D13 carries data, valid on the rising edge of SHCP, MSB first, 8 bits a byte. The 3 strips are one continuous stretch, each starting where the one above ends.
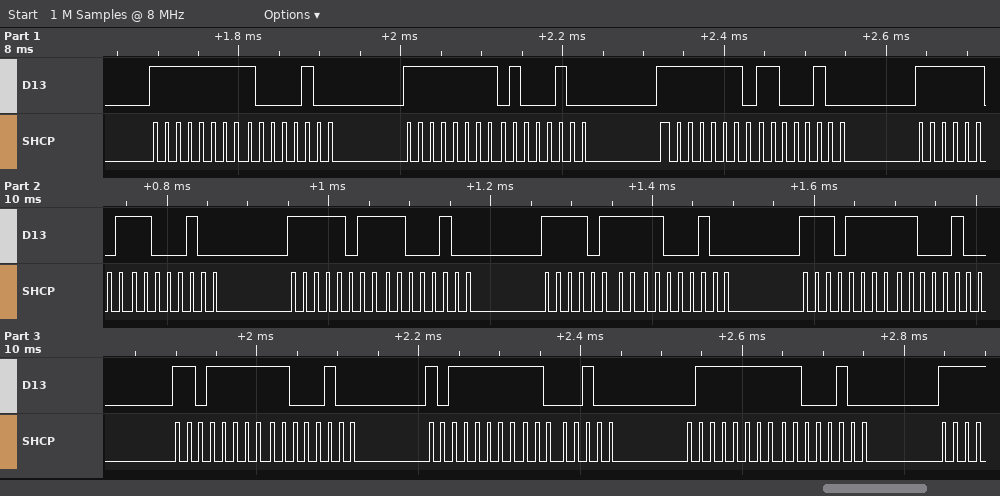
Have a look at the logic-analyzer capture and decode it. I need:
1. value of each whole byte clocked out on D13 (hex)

FF 84 FF 44 FE C4 FD C4 FB C4 F7 C4 EF C4 DF C4 BF C4 7F C4
